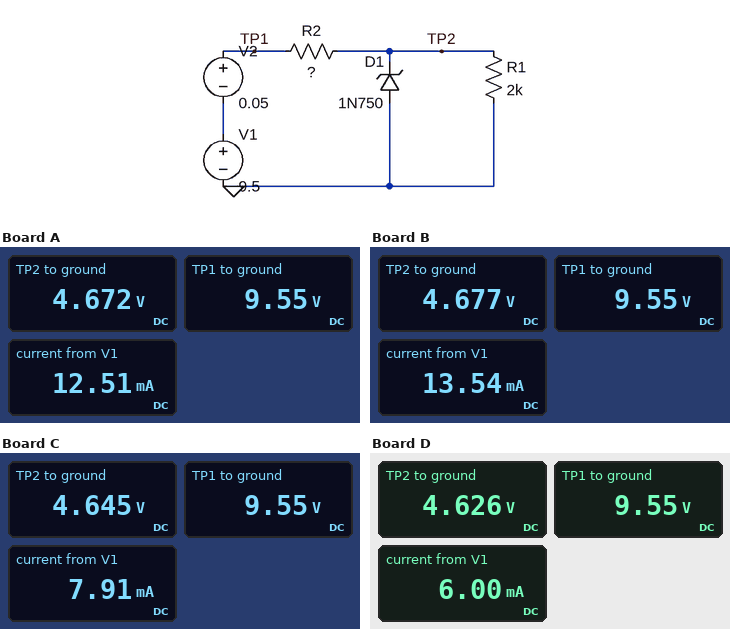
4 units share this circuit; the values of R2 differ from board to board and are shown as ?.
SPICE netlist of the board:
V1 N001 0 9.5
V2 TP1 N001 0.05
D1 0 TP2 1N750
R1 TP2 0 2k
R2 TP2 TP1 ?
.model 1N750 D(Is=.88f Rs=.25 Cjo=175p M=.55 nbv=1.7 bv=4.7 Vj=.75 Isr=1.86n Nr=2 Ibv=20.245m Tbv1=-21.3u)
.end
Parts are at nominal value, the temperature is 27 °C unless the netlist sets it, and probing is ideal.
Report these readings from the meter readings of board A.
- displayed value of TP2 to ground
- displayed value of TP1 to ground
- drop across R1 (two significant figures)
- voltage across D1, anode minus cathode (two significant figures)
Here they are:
4.672 V
9.55 V
4.7 V
-4.7 V
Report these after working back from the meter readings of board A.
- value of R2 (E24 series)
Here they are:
390 Ω
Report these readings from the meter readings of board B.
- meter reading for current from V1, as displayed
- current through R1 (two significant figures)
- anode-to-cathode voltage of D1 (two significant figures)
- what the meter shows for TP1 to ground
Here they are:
13.54 mA
2.3 mA
-4.7 V
9.55 V
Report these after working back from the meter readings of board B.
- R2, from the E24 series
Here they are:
360 Ω
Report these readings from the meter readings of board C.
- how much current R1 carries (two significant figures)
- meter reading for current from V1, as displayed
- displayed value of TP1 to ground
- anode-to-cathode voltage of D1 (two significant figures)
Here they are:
2.3 mA
7.91 mA
9.55 V
-4.6 V
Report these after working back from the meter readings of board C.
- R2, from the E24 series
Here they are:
620 Ω
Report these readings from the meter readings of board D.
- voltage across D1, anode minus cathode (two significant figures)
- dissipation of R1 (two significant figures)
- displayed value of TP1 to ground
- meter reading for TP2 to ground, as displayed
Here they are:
-4.6 V
11 mW
9.55 V
4.626 V
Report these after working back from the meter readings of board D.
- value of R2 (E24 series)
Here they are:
820 Ω
